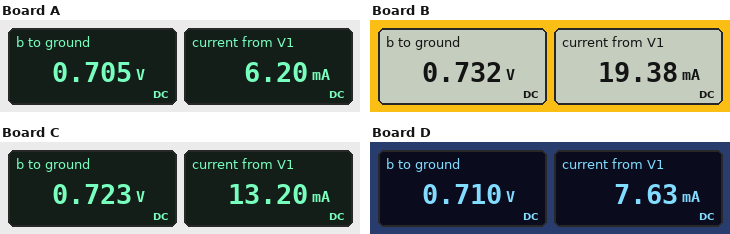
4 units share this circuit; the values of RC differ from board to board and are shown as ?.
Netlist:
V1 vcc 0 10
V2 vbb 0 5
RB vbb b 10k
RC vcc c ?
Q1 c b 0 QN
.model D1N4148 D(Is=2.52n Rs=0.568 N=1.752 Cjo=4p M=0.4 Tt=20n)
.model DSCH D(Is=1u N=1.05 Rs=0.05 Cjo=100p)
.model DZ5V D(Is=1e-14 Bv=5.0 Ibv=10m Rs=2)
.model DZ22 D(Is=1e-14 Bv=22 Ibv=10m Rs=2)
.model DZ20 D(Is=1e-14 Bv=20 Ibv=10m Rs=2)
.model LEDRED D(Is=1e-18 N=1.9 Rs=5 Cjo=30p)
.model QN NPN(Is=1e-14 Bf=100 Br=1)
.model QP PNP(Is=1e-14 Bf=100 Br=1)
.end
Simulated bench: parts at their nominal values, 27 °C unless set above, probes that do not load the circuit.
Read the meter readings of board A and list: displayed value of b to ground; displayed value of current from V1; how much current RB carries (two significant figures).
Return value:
0.705 V
6.20 mA
430 µA
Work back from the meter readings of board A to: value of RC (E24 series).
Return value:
1.6 kΩ
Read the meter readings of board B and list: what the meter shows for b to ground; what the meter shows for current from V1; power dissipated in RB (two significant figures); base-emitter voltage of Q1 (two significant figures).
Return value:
0.732 V
19.38 mA
1.8 mW
730 mV
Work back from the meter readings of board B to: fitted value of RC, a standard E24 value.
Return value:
510 Ω
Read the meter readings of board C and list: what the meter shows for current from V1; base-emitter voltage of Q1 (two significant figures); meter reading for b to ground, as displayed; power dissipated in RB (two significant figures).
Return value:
13.20 mA
720 mV
0.723 V
1.8 mW
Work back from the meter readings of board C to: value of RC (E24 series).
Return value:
750 Ω
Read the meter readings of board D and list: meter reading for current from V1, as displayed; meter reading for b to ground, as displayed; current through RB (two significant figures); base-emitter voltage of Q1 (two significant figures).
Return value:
7.63 mA
0.710 V
430 µA
710 mV
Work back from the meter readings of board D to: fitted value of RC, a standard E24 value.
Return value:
1.3 kΩ
